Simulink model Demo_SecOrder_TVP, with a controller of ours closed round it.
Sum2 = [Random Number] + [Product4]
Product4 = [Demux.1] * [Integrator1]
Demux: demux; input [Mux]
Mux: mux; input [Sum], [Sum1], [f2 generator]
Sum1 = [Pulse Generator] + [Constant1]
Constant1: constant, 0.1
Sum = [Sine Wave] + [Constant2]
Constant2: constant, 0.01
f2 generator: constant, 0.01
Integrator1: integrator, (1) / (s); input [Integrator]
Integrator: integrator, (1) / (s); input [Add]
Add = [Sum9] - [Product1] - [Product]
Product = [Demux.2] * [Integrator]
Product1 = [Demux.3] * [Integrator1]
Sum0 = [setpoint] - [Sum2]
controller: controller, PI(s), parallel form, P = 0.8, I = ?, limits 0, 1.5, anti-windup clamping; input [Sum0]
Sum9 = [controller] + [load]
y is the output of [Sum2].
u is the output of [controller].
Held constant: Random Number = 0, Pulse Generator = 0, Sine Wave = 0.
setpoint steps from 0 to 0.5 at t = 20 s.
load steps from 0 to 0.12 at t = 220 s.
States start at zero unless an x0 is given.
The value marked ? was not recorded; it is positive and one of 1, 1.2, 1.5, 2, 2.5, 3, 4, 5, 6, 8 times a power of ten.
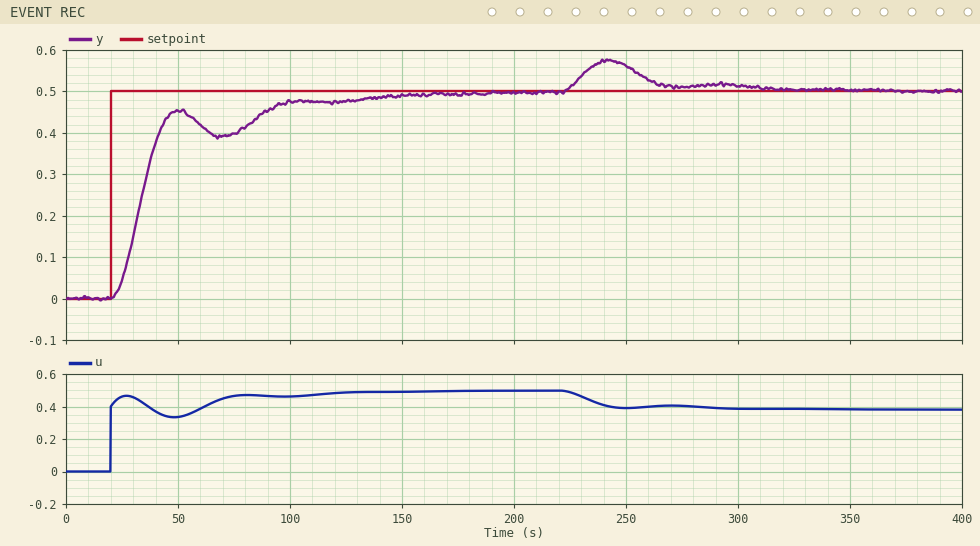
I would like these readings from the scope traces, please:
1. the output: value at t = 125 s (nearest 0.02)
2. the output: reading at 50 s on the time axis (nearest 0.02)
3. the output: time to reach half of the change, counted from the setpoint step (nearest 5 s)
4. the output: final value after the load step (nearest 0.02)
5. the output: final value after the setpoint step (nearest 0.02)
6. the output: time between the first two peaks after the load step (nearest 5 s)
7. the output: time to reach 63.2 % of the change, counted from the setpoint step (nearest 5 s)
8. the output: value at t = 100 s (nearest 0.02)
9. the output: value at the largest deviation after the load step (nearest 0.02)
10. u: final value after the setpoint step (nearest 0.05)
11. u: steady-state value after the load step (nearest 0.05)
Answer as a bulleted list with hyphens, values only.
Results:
- 0.48
- 0.46
- 15 s
- 0.50
- 0.50
- 50 s
- 15 s
- 0.48
- 0.58
- 0.50
- 0.40
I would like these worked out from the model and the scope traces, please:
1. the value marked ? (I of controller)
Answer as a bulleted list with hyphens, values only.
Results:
- 0.04
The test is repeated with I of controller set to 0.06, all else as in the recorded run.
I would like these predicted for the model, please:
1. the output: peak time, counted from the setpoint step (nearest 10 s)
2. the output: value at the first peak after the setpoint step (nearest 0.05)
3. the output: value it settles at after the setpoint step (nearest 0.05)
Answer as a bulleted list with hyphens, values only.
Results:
- 30 s
- 0.55
- 0.50
